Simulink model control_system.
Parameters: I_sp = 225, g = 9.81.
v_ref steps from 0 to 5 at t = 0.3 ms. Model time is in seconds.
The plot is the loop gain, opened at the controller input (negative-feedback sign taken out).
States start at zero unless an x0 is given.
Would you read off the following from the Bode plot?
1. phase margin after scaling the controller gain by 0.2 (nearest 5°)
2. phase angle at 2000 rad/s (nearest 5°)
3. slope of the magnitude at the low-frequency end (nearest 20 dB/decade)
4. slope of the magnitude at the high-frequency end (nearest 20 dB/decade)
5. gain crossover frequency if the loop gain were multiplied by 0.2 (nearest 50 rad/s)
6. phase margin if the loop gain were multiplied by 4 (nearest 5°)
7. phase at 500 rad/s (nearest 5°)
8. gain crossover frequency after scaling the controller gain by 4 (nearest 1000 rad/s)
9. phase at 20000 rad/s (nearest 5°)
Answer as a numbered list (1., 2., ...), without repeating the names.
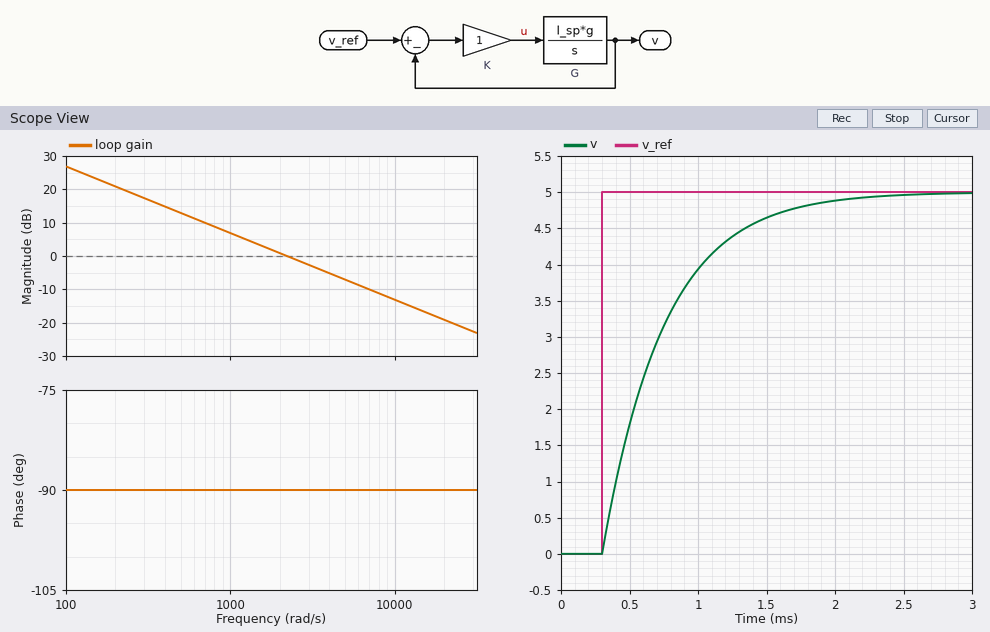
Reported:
1. 90°
2. -90°
3. -20 dB/decade
4. -20 dB/decade
5. 450 rad/s
6. 90°
7. -90°
8. 9000 rad/s
9. -90°
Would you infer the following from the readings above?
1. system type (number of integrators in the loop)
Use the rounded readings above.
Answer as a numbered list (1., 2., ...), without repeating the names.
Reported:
1. 1
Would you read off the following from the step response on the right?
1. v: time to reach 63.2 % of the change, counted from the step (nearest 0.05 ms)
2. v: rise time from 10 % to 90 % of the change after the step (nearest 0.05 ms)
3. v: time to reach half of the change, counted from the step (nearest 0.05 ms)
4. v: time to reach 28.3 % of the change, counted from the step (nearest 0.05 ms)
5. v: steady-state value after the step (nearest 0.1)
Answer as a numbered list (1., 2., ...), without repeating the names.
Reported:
1. 0.45 ms
2. 1.00 ms
3. 0.30 ms
4. 0.15 ms
5. 5.0
